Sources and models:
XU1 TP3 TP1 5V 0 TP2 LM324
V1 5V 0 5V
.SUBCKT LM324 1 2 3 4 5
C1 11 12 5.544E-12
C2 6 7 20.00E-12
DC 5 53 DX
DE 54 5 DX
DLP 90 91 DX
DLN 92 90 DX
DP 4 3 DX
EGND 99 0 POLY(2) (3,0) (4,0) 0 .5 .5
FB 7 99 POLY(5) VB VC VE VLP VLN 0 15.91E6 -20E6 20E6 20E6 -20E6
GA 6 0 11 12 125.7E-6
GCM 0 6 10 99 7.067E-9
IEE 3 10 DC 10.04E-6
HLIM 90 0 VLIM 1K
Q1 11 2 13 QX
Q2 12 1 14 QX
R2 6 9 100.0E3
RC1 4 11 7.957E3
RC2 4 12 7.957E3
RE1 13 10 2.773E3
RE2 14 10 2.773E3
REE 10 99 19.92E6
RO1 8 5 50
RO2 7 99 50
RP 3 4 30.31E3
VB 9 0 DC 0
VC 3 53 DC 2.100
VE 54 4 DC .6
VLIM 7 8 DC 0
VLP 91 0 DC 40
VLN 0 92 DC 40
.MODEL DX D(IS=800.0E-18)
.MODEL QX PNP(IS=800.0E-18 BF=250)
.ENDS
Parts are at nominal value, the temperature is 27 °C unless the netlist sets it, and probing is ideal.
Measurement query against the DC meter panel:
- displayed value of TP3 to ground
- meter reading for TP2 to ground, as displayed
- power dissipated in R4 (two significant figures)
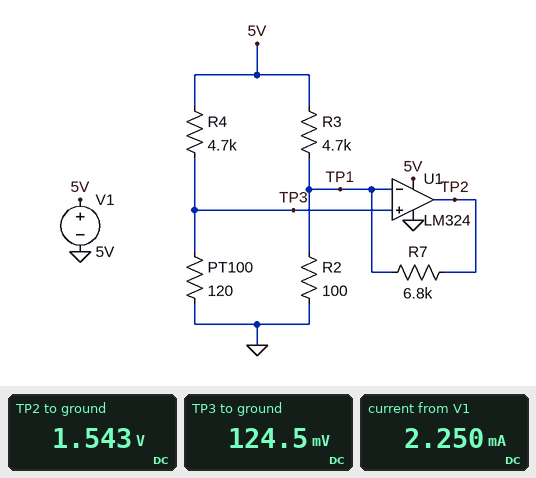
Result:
124.5 mV
1.543 V
5.1 mW
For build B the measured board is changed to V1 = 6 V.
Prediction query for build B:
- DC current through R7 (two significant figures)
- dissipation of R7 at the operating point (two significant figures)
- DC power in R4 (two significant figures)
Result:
250 µA
430 µW
7.3 mW
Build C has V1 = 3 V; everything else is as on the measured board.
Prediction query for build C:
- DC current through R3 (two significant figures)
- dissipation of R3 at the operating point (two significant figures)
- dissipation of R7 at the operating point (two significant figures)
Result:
620 µA
1.8 mW
110 µW
